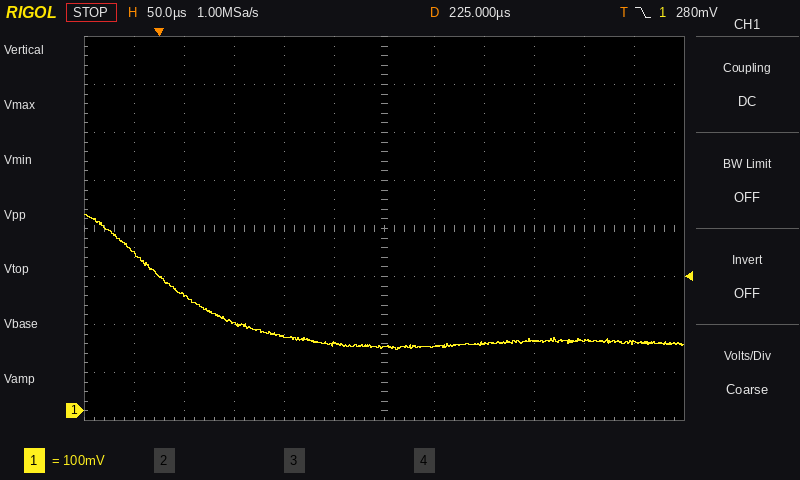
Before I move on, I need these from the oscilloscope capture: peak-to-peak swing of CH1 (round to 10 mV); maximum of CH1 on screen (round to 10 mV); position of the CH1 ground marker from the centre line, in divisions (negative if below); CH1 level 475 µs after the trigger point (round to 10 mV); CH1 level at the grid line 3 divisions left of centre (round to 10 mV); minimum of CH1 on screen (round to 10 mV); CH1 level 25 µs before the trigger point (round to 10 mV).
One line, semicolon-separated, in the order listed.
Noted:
280 mV; 410 mV; -3.8 div; 140 mV; 180 mV; 130 mV; 330 mV
